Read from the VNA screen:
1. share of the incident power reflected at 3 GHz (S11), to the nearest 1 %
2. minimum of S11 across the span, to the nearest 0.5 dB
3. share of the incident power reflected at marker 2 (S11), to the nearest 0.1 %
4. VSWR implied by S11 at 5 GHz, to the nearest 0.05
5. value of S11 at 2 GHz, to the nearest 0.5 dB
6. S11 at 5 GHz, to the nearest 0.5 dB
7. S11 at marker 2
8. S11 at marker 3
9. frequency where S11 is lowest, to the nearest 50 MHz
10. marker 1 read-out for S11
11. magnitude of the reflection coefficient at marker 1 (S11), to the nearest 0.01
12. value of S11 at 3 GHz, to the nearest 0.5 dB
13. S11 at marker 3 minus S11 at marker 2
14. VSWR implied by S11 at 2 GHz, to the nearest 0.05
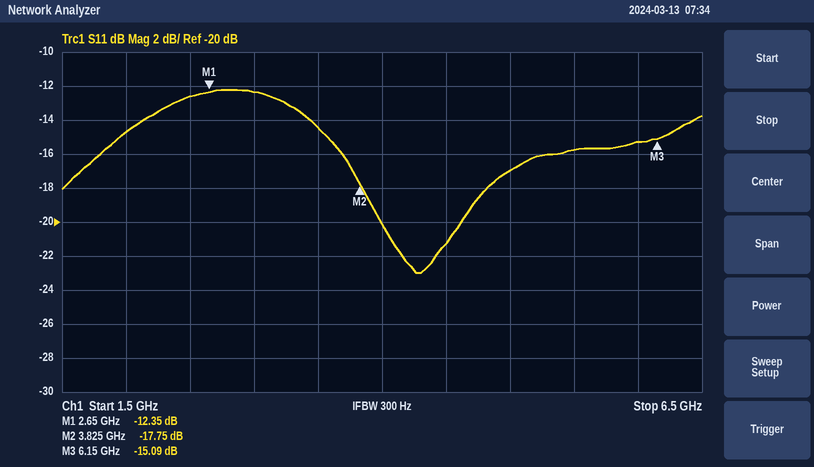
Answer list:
6 %
-23.0 dB
1.7 %
1.35
-14.5 dB
-17.0 dB
-17.75 dB
-15.09 dB
4.25 GHz
-12.35 dB
0.24
-12.5 dB
2.66 dB
1.45
